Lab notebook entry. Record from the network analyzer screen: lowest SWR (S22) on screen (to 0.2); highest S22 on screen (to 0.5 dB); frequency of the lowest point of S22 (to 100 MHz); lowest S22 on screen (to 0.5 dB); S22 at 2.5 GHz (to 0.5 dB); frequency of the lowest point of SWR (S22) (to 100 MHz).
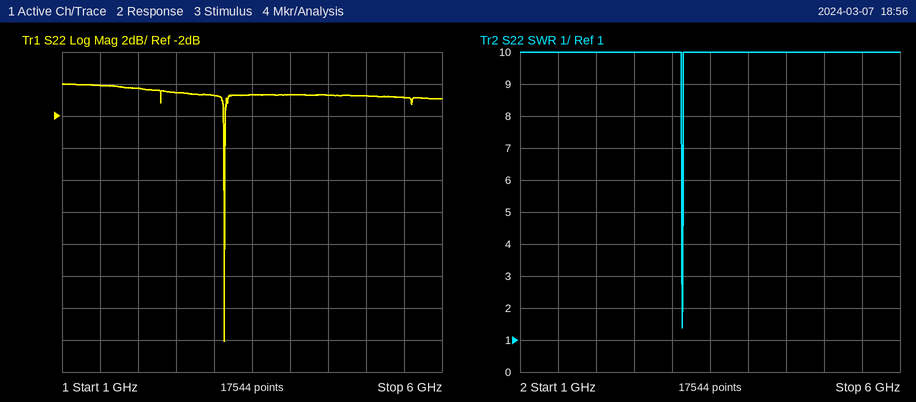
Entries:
1.4
0.0 dB
3.1 GHz
-16.0 dB
-0.5 dB
3.1 GHz
